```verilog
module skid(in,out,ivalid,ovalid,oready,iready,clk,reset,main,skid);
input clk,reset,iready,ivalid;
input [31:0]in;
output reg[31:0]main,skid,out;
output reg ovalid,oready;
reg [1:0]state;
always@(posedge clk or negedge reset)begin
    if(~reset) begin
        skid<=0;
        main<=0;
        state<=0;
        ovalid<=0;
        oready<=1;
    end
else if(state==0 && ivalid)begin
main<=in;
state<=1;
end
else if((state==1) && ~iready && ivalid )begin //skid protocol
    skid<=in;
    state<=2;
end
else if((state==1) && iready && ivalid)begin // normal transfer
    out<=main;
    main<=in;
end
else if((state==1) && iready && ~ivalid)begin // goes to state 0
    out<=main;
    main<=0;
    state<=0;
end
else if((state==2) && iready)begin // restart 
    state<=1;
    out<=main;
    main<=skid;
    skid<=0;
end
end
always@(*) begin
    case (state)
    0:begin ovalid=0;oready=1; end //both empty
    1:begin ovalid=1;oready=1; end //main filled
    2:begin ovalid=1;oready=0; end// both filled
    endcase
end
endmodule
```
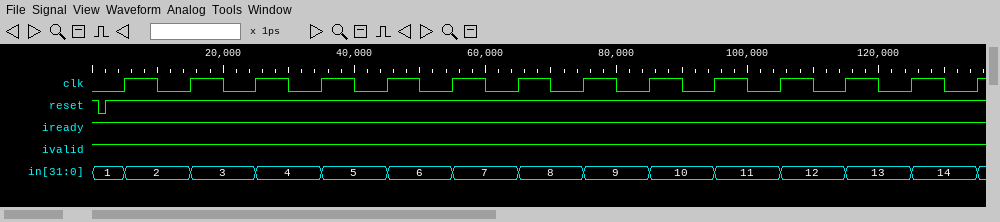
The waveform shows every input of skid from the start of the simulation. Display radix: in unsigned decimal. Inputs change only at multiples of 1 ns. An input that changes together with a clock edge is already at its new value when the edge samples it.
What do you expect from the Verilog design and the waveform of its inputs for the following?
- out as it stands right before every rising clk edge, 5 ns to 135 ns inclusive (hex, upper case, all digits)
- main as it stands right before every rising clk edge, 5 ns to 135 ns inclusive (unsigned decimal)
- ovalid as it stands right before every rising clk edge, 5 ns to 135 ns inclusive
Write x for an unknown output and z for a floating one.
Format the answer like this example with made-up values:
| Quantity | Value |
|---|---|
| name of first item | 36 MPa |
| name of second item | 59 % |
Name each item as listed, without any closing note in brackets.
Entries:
| Quantity | Value |
|---|---|
| out as it stands right before every rising clk edge, 5 ns to 135 ns inclusive | x, x, 00000002, 00000003, 00000004, 00000005, 00000006, 00000007, 00000008, 00000009, 0000000A, 0000000B, 0000000C, 0000000D |
| main as it stands right before every rising clk edge, 5 ns to 135 ns inclusive | 0, 2, 3, 4, 5, 6, 7, 8, 9, 10, 11, 12, 13, 14 |
| ovalid as it stands right before every rising clk edge, 5 ns to 135 ns inclusive | 0 1 1 1 1 1 1 1 1 1 1 1 1 1 |
